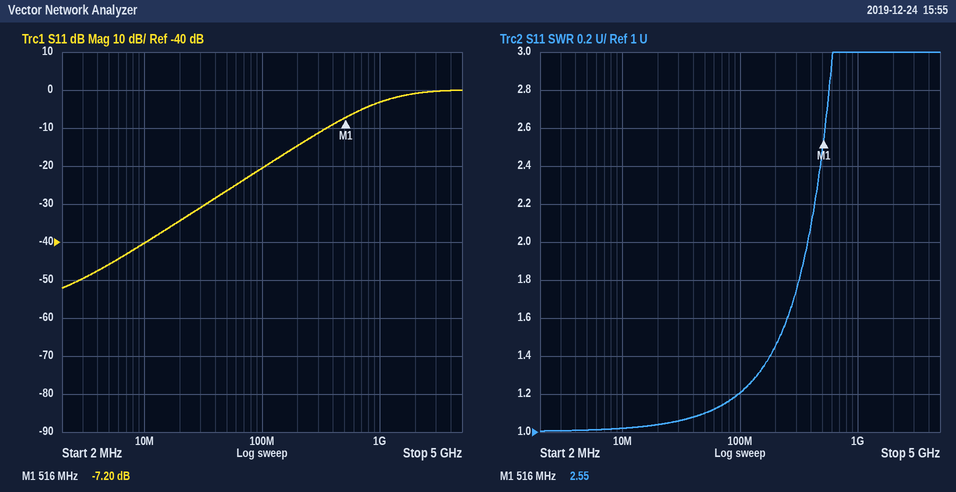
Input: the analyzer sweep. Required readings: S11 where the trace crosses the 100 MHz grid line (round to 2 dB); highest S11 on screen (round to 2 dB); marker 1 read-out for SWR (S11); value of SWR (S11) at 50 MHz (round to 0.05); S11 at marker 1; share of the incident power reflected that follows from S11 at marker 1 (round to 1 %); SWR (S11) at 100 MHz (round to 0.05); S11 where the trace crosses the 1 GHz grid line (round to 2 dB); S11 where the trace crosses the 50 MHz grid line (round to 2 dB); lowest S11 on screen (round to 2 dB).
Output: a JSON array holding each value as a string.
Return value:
["-20 dB", "0 dB", "2.55", "1.10", "-7.20 dB", "19 %", "1.20", "-4 dB", "-26 dB", "-52 dB"]
